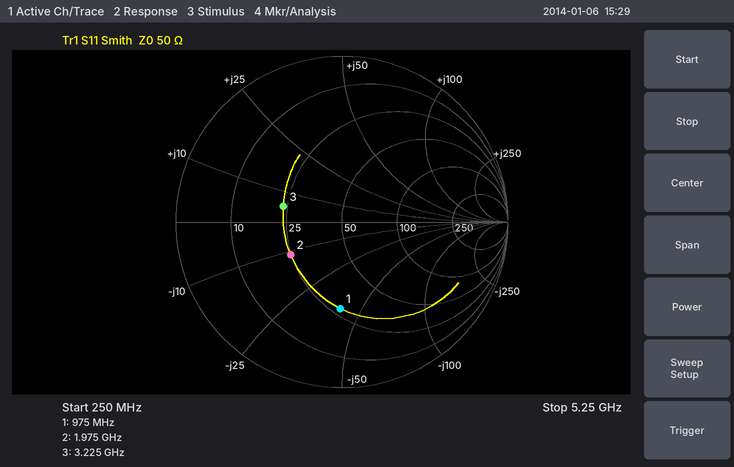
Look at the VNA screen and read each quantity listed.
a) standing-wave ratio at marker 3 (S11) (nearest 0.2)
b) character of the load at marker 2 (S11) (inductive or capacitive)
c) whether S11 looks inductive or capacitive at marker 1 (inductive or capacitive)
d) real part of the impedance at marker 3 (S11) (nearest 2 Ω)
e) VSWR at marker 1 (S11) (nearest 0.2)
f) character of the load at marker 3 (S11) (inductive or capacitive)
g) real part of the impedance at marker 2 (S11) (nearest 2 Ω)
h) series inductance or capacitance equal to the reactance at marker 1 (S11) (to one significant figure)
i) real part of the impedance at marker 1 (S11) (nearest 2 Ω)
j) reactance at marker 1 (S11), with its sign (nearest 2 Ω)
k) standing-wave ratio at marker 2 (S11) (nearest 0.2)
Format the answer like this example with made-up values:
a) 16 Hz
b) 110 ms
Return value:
a) 2.2
b) capacitive
c) capacitive
d) 24 Ω
e) 3.2
f) inductive
g) 24 Ω
h) 4 pF
i) 28 Ω
j) -40 Ω
k) 2.2
